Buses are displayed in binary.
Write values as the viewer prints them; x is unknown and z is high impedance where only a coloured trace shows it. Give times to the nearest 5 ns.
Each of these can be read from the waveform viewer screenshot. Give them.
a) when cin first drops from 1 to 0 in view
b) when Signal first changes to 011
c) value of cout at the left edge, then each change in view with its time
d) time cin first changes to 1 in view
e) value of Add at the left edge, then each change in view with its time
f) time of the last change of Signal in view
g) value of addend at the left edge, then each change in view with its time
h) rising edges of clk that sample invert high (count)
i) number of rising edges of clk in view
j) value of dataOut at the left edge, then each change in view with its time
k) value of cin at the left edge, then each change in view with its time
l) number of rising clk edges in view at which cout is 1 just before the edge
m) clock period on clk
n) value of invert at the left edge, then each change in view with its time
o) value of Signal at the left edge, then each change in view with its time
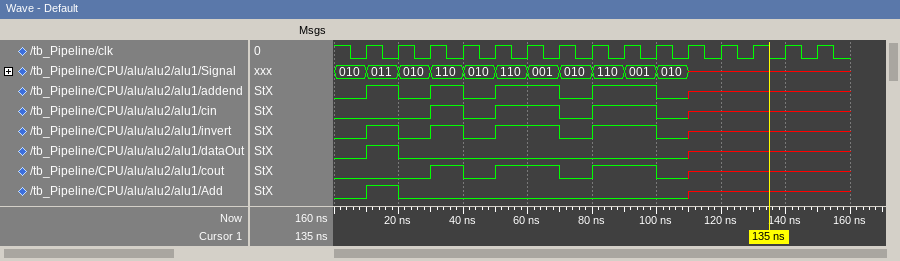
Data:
40 ns
10 ns
0, 1 at 30 ns, 0 at 40 ns, 1 at 50 ns, 0 at 70 ns, 1 at 80 ns, 0 at 100 ns, x at 110 ns
30 ns
0, 1 at 10 ns, 0 at 20 ns, x at 110 ns
110 ns
0, 1 at 10 ns, 0 at 20 ns, 1 at 30 ns, 0 at 40 ns, 1 at 50 ns, 0 at 70 ns, 1 at 80 ns, 0 at 100 ns, x at 110 ns
6
15
0, 1 at 10 ns, 0 at 20 ns, x at 110 ns
0, 1 at 30 ns, 0 at 40 ns, 1 at 50 ns, 0 at 70 ns, 1 at 80 ns, 0 at 100 ns, x at 110 ns
5
10 ns
0, 1 at 10 ns, 0 at 20 ns, 1 at 30 ns, 0 at 40 ns, 1 at 50 ns, 0 at 70 ns, 1 at 80 ns, 0 at 100 ns, x at 110 ns
010, 011 at 10 ns, 010 at 20 ns, 110 at 30 ns, 010 at 40 ns, 110 at 50 ns, 001 at 60 ns, 010 at 70 ns, 110 at 80 ns, 001 at 90 ns, 010 at 100 ns, x at 110 ns
